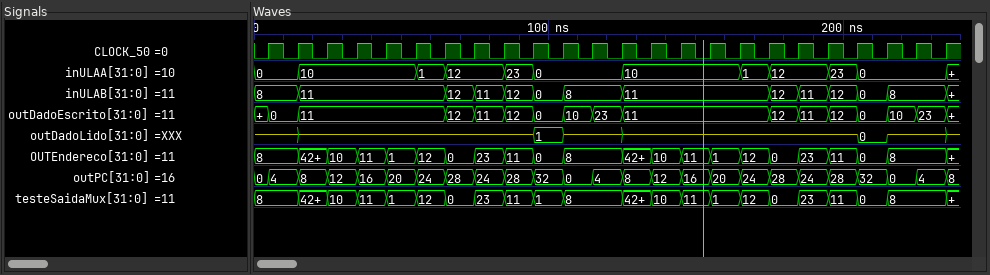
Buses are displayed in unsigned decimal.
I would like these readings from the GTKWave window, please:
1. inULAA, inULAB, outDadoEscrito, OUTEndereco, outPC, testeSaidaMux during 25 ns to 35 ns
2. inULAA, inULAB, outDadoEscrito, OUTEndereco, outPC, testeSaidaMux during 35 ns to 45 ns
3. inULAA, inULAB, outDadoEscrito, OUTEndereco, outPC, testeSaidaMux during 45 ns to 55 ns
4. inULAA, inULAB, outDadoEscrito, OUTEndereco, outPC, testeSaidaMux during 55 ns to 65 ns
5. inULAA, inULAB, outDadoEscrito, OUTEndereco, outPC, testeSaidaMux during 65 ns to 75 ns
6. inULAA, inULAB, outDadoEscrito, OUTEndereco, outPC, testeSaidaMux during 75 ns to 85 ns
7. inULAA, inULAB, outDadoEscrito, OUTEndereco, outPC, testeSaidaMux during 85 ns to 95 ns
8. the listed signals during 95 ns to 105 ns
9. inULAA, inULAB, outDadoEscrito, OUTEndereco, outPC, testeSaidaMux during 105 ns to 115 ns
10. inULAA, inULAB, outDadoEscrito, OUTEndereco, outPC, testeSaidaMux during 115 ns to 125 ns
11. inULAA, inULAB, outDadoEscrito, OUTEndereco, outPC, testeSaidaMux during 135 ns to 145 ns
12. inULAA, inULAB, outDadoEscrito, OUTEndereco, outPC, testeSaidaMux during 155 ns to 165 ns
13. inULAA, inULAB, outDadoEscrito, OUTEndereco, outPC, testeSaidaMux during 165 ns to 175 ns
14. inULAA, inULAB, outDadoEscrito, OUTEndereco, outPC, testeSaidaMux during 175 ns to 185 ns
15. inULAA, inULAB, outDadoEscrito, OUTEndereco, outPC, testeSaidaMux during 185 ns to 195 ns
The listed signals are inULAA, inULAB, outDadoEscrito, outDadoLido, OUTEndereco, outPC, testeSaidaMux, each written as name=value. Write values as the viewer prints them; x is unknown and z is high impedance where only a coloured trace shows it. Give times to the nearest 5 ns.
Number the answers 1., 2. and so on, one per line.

1. inULAA=10, inULAB=11, outDadoEscrito=11, OUTEndereco=10, outPC=12, testeSaidaMux=10
2. inULAA=10, inULAB=11, outDadoEscrito=11, OUTEndereco=11, outPC=16, testeSaidaMux=11
3. inULAA=10, inULAB=11, outDadoEscrito=11, OUTEndereco=1, outPC=20, testeSaidaMux=1
4. inULAA=1, inULAB=11, outDadoEscrito=11, OUTEndereco=12, outPC=24, testeSaidaMux=12
5. inULAA=12, inULAB=12, outDadoEscrito=12, OUTEndereco=0, outPC=28, testeSaidaMux=0
6. inULAA=12, inULAB=11, outDadoEscrito=11, OUTEndereco=23, outPC=24, testeSaidaMux=23
7. inULAA=23, inULAB=12, outDadoEscrito=12, OUTEndereco=11, outPC=28, testeSaidaMux=11
8. inULAA=0, inULAB=0, outDadoEscrito=0, outDadoLido=1, OUTEndereco=0, outPC=32, testeSaidaMux=1
9. inULAA=0, inULAB=8, outDadoEscrito=10, OUTEndereco=8, outPC=0, testeSaidaMux=8
10. inULAA=0, inULAB=8, outDadoEscrito=23, OUTEndereco=8, outPC=4, testeSaidaMux=8
11. inULAA=10, inULAB=11, outDadoEscrito=11, OUTEndereco=10, outPC=12, testeSaidaMux=10
12. inULAA=10, inULAB=11, outDadoEscrito=11, OUTEndereco=1, outPC=20, testeSaidaMux=1
13. inULAA=1, inULAB=11, outDadoEscrito=11, OUTEndereco=12, outPC=24, testeSaidaMux=12
14. inULAA=12, inULAB=12, outDadoEscrito=12, OUTEndereco=0, outPC=28, testeSaidaMux=0
15. inULAA=12, inULAB=11, outDadoEscrito=11, OUTEndereco=23, outPC=24, testeSaidaMux=23
